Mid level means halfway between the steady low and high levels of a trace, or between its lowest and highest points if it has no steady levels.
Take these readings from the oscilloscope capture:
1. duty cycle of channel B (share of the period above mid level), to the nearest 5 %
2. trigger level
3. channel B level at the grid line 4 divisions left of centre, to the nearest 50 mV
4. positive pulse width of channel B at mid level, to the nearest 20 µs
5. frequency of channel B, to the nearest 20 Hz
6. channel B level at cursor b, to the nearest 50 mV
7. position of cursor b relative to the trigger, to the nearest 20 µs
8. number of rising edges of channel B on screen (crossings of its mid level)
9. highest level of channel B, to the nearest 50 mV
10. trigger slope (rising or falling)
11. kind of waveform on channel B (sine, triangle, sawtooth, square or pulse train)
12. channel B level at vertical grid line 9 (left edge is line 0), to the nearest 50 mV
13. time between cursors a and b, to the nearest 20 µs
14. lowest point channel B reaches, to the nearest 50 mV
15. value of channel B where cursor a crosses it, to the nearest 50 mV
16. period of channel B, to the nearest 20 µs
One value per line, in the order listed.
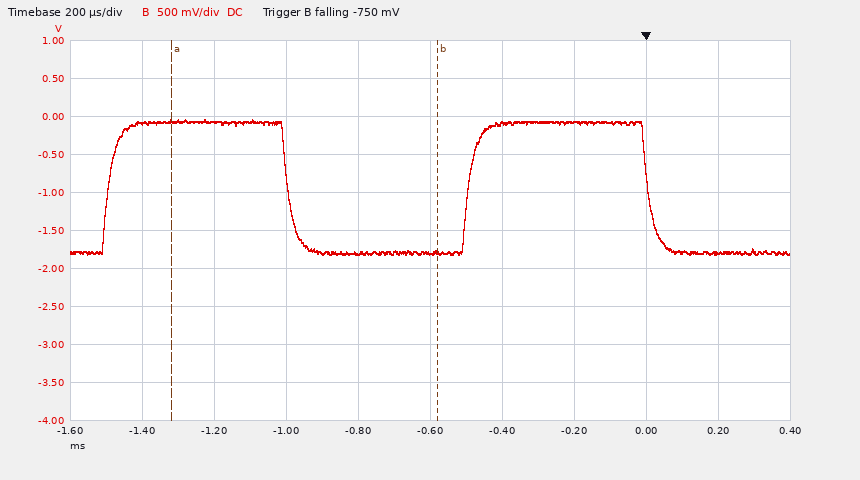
50 %
-750 mV
-100 mV
500 µs
1.00 kHz
-1.80 V
-580 µs
2
-50 mV
falling
square
-1.80 V
740 µs
-1.80 V
-50 mV
1.00 ms
